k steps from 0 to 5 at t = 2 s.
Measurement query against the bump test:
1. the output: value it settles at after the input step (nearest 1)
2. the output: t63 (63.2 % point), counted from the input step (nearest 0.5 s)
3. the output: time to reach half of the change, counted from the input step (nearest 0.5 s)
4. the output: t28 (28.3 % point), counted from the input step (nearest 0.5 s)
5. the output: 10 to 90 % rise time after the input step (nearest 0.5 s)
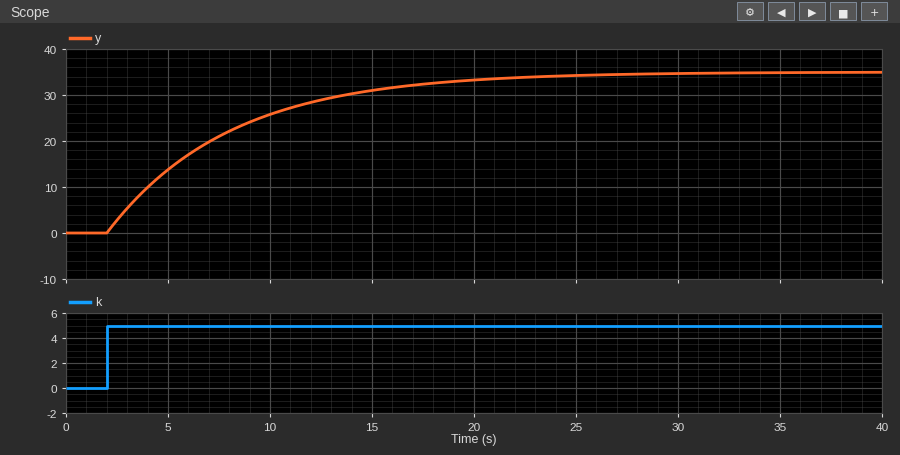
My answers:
35
6.0 s
4.0 s
2.0 s
13.0 s
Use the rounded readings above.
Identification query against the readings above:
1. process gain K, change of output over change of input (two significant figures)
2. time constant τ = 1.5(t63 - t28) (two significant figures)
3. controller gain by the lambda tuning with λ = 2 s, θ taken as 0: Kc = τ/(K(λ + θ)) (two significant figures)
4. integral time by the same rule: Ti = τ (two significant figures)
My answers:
7.0
6.0 s
0.43
6.0 s
